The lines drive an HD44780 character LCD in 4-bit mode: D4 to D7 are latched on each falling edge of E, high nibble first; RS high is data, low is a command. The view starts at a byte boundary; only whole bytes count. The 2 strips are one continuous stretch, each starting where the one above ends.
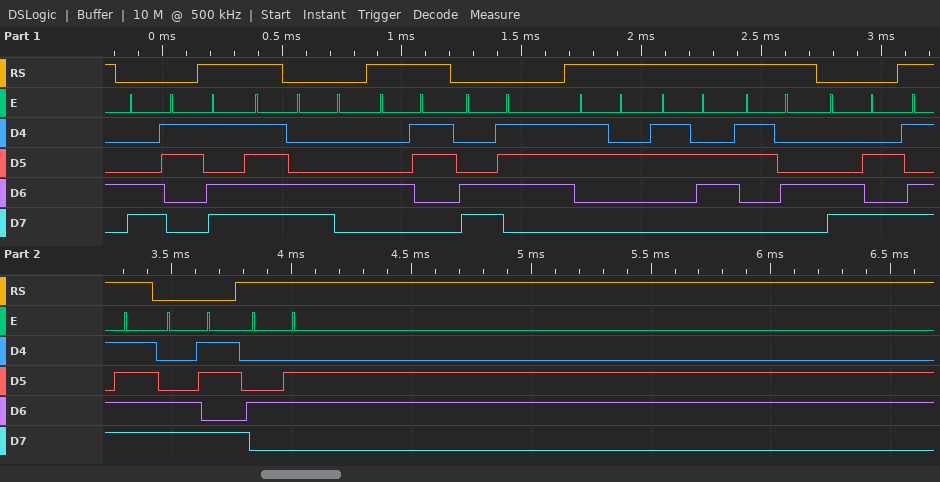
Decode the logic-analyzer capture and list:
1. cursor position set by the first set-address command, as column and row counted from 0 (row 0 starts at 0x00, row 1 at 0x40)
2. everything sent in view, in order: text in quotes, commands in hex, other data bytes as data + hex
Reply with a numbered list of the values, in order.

1. column 3, row 1
2. 0xC3 data DF 0xC4 "C" 0xC7 "264" 0xCA data DF 0xCB "F"
